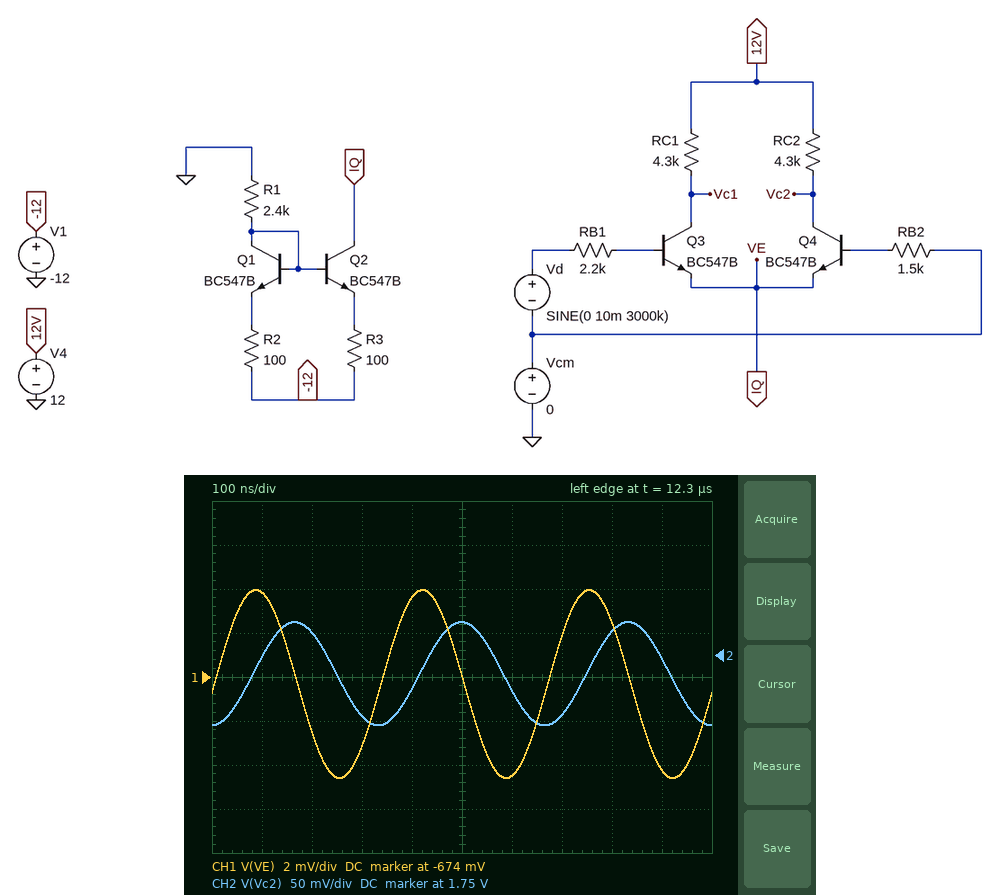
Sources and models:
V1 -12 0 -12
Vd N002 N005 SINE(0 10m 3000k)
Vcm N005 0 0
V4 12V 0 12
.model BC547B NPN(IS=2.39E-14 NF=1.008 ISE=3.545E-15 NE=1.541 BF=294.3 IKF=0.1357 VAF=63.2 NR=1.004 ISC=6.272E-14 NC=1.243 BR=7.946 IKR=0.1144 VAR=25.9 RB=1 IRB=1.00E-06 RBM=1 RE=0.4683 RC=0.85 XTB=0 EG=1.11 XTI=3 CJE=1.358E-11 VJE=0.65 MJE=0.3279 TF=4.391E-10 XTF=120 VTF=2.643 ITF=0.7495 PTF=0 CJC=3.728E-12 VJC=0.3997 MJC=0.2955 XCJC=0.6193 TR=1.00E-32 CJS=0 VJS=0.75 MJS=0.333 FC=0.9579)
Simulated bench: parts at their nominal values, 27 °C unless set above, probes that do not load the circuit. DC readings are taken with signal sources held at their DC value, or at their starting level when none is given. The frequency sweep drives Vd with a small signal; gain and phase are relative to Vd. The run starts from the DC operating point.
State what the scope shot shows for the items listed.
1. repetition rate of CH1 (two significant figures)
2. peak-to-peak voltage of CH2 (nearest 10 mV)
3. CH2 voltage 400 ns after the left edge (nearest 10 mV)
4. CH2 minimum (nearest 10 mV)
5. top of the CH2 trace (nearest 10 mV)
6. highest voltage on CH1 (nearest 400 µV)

3.0 MHz
120 mV
1.71 V
1.67 V
1.79 V
-670.0 mV
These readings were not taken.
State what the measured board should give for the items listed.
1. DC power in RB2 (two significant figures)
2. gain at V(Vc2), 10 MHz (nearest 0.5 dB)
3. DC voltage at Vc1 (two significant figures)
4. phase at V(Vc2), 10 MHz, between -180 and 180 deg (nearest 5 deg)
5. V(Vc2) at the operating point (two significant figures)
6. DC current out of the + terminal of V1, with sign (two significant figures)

100 nW
4.5 dB
2.8 V
-95 deg
1.7 V
-9.1 mA
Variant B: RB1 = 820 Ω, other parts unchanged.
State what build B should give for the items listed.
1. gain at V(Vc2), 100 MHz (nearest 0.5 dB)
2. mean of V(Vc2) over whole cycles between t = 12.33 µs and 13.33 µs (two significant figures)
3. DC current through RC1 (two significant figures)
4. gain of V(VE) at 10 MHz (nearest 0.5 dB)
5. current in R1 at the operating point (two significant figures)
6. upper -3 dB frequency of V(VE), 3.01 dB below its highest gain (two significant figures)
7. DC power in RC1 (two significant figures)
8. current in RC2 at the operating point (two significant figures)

-10.5 dB
2.9 V
2.4 mA
-4.5 dB
4.5 mA
72 MHz
25 mW
2.1 mA
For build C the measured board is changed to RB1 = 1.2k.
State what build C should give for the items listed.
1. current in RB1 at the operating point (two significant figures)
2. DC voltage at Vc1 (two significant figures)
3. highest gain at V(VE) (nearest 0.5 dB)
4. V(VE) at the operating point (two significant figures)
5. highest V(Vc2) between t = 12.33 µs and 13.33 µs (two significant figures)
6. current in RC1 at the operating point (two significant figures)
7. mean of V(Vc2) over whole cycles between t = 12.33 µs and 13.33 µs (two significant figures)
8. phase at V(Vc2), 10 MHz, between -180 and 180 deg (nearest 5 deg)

8.0 µA
2.0 V
-5.5 dB
-670 mV
2.6 V
2.3 mA
2.5 V
-90 deg
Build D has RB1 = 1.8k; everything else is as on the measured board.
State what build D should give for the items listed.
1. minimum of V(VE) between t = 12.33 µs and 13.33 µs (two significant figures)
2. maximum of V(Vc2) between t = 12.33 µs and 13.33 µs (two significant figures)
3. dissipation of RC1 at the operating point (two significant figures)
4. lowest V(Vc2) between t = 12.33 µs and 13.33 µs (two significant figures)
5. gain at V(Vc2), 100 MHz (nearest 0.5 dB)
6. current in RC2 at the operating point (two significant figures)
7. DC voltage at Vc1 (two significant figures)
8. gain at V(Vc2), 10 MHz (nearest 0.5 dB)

-680 mV
2.1 V
21 mW
2.0 V
-15.5 dB
2.3 mA
2.5 V
5.5 dB
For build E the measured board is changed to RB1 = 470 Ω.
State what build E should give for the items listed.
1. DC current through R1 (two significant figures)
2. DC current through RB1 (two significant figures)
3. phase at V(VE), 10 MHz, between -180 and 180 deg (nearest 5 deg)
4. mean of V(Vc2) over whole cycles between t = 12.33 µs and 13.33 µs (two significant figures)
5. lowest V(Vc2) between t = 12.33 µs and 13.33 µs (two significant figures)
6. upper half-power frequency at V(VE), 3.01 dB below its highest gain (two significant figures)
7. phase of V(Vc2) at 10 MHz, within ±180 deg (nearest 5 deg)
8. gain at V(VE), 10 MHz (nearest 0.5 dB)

4.5 mA
8.7 µA
-5 deg
3.2 V
3.1 V
130 MHz
-85 deg
-3.0 dB
